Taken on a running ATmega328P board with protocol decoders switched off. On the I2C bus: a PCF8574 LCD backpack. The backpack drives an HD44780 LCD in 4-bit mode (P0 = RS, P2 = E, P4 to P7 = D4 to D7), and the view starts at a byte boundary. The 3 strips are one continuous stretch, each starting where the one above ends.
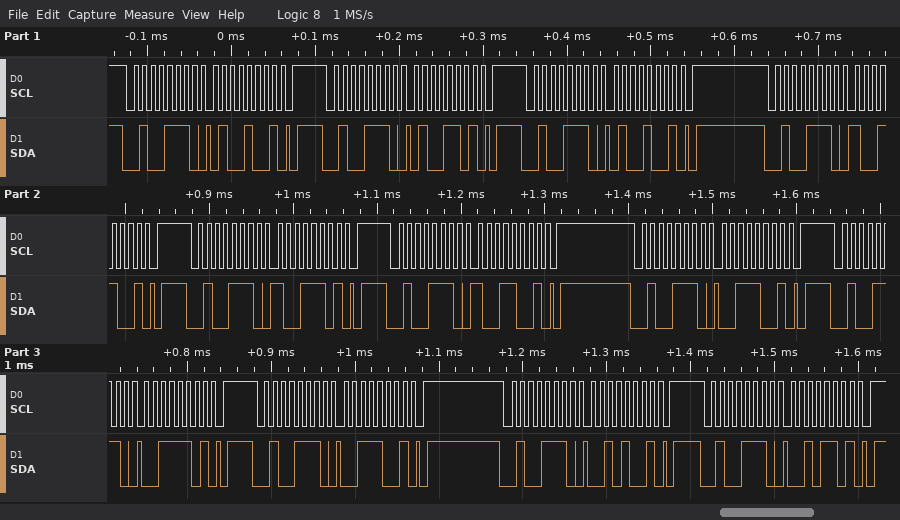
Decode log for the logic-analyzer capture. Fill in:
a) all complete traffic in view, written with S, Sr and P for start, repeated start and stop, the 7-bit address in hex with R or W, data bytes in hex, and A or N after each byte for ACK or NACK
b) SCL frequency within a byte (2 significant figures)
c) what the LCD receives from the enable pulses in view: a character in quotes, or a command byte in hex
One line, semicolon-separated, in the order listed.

S 27W A 49 A P S 27W A 4D A P S 27W A 49 A P S 27W A 99 A P S 27W A 9D A P S 27W A 99 A P S 27W A 39 A P S 27W A 3D A P S 27W A 39 A P S 27W A 29 A P S 27W A 2D A P; 100 kHz; 'I'
